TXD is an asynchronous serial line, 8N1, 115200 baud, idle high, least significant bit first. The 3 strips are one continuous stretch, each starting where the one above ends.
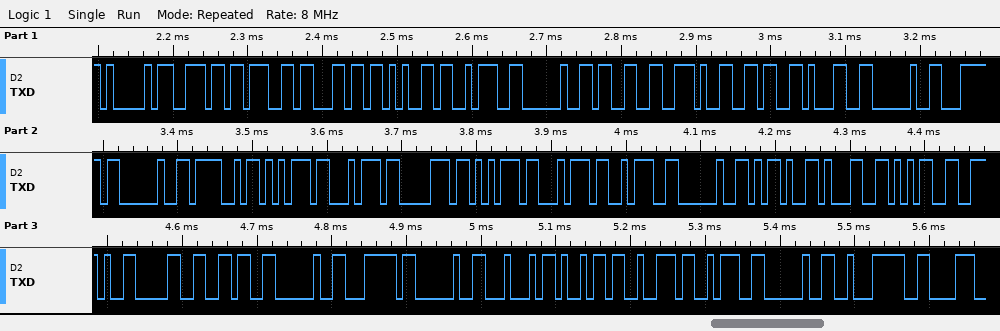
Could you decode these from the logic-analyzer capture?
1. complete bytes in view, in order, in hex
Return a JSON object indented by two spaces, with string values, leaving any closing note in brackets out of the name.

{
  "complete bytes in view, in order, in hex": "41 6E 67 6C 65 3A 20 33 2E 36 31 20 7C 20 4F 75 74 70 75 74 3A 20 2D 31 35 2E 30 36 20 7C 20 44 69 72 3A 20 E2 86"
}
